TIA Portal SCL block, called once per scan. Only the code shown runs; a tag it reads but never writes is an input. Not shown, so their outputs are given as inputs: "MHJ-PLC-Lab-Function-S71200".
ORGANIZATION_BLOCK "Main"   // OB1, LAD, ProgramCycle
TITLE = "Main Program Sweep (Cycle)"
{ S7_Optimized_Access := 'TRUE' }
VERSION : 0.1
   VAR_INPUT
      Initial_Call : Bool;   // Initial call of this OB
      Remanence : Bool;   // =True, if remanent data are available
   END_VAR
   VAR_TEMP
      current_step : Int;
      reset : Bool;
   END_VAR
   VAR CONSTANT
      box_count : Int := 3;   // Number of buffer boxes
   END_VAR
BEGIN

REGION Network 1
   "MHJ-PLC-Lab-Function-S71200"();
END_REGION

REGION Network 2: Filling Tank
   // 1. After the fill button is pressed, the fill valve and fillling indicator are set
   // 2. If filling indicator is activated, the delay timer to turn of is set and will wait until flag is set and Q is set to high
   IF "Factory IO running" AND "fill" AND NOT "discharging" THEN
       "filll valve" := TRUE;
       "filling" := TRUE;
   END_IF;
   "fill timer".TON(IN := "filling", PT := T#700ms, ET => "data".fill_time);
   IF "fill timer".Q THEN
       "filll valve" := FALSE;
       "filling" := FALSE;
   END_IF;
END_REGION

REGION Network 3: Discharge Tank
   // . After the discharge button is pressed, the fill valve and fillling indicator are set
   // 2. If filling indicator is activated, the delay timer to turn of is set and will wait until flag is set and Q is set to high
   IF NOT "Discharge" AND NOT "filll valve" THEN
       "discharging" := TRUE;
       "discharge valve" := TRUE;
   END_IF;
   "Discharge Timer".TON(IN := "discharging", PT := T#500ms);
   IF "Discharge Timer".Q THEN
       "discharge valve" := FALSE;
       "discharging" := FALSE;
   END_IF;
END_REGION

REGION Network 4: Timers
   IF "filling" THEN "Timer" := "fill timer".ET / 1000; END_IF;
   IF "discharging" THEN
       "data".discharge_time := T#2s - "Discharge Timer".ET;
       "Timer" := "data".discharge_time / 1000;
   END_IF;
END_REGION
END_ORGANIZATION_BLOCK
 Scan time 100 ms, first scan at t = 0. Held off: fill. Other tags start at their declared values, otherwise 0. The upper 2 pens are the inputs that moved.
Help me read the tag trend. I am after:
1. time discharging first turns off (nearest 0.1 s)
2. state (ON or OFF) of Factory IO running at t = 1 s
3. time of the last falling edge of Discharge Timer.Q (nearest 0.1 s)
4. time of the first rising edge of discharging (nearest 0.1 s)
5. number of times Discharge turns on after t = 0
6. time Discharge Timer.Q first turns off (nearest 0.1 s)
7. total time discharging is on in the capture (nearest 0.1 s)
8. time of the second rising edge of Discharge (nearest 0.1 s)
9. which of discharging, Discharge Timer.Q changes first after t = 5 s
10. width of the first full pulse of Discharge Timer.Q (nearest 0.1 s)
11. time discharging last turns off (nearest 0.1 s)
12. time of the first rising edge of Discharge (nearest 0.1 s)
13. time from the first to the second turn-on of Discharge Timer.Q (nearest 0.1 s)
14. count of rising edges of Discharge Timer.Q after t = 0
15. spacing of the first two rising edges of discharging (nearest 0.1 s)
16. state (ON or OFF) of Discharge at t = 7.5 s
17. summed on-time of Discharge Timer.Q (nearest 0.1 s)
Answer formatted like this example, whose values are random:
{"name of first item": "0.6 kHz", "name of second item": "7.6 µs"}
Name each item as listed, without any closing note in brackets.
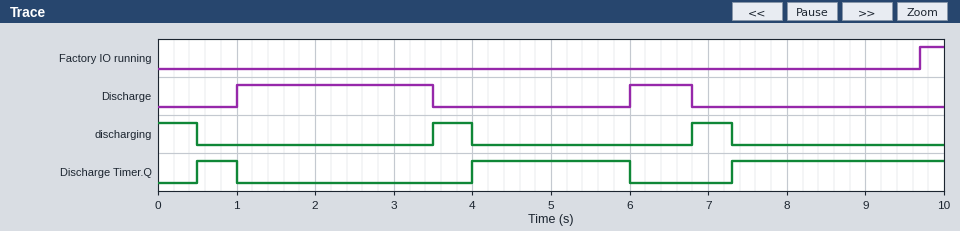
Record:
{"time discharging first turns off": "0.5 s", "state (ON or OFF) of Factory IO running at t = 1 s": "OFF", "time of the last falling edge of Discharge Timer.Q": "6.0 s", "time of the first rising edge of discharging": "3.5 s", "number of times Discharge turns on after t = 0": "2", "time Discharge Timer.Q first turns off": "1.0 s", "total time discharging is on in the capture": "1.5 s", "time of the second rising edge of Discharge": "6.0 s", "which of discharging, Discharge Timer.Q changes first after t = 5 s": "Discharge Timer.Q", "width of the first full pulse of Discharge Timer.Q": "0.5 s", "time discharging last turns off": "7.3 s", "time of the first rising edge of Discharge": "1.0 s", "time from the first to the second turn-on of Discharge Timer.Q": "3.5 s", "count of rising edges of Discharge Timer.Q after t = 0": "3", "spacing of the first two rising edges of discharging": "3.3 s", "state (ON or OFF) of Discharge at t = 7.5 s": "OFF", "summed on-time of Discharge Timer.Q": "5.2 s"}
